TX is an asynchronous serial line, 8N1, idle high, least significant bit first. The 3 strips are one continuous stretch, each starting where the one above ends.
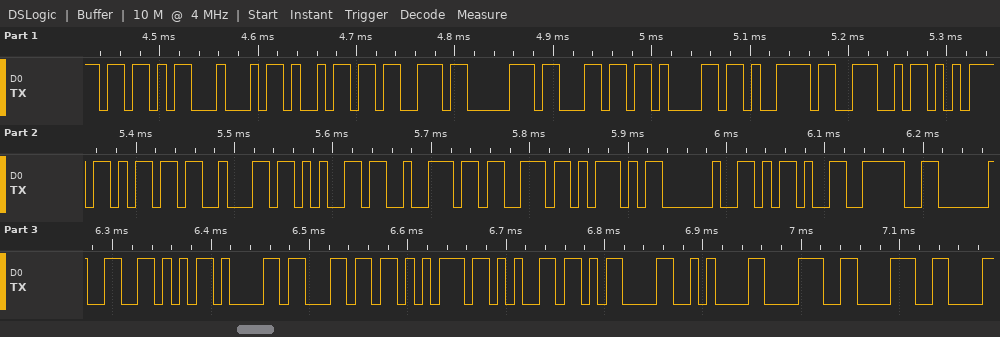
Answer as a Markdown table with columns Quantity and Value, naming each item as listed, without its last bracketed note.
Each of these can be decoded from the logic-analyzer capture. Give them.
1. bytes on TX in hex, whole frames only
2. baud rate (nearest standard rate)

| Quantity | Value |
|---|---|
| bytes on TX in hex, whole frames only | 5B 44 69 73 70 6C 61 79 4E 75 6D 62 65 72 73 5D 20 2D 3E 20 56 61 6C 75 65 0D 0A 38 38 |
| baud rate | 115200 baud |
